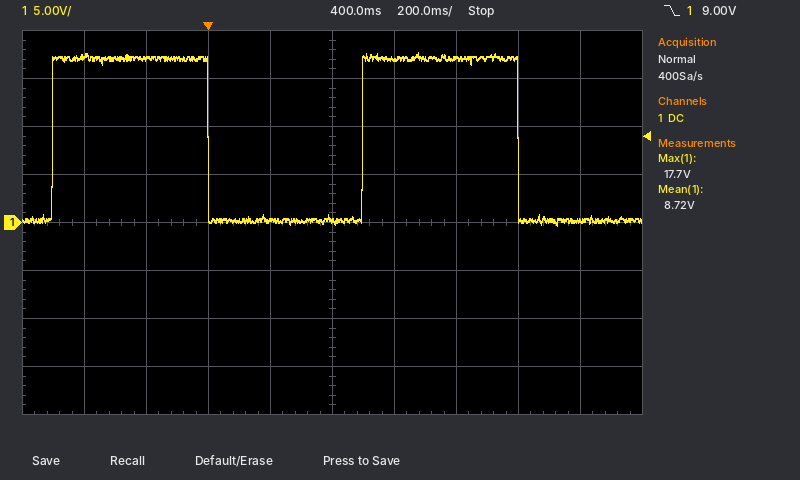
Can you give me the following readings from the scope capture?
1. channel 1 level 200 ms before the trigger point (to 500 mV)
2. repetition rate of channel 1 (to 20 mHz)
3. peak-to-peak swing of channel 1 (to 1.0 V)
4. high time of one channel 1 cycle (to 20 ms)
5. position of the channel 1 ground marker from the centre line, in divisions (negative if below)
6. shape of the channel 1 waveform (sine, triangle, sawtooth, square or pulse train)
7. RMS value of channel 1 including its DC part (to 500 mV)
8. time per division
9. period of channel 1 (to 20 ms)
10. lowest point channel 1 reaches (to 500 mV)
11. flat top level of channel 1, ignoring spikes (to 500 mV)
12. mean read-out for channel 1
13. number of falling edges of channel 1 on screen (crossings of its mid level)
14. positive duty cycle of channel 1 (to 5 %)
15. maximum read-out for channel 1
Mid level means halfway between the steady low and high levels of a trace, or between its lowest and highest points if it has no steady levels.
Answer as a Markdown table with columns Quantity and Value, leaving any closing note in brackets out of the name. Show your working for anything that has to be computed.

| Quantity | Value |
|---|---|
| channel 1 level 200 ms before the trigger point | 17.0 V |
| repetition rate of channel 1 | 1 / 1.00 s ≈ 1.00 Hz |
| peak-to-peak swing of channel 1 | 18.0 V |
| high time of one channel 1 cycle | 500 ms |
| position of the channel 1 ground marker from the centre line, in divisions | 0.0 div |
| shape of the channel 1 waveform | square |
| RMS value of channel 1 including its DC part | √(0.5 × (17.0 V)² + 0.5 × (-500 mV)²) ≈ 12.0 V |
| time per division | 200 ms |
| period of channel 1 | 1.00 s |
| lowest point channel 1 reaches | -500 mV |
| flat top level of channel 1, ignoring spikes | 17.0 V |
| mean read-out for channel 1 | 8.72 V |
| number of falling edges of channel 1 on screen | 2 |
| positive duty cycle of channel 1 | 500 ms / 1.00 s ≈ 50 % |
| maximum read-out for channel 1 | 17.7 V |
